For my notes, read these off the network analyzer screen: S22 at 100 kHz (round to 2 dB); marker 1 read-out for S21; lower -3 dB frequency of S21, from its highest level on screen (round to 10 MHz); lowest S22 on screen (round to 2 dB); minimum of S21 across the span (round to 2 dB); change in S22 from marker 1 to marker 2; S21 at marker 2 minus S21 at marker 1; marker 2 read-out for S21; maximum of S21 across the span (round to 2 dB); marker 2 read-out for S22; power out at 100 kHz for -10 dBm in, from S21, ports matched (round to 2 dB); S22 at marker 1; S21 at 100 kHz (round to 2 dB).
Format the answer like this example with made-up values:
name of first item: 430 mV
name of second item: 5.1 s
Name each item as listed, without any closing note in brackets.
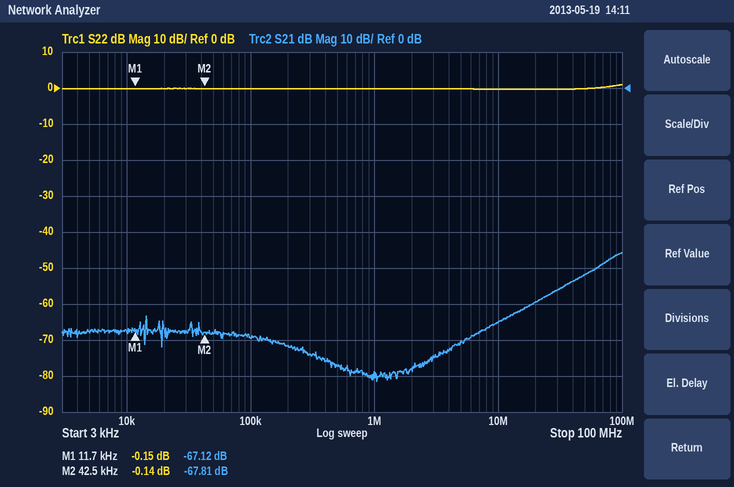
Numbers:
S22 at 100 kHz: 0 dB
marker 1 read-out for S21: -67.12 dB
lower -3 dB frequency of S21, from its highest level on screen: 70 MHz
lowest S22 on screen: 0 dB
minimum of S21 across the span: -82 dB
change in S22 from marker 1 to marker 2: 0.01 dB
S21 at marker 2 minus S21 at marker 1: -0.69 dB
marker 2 read-out for S21: -67.81 dB
maximum of S21 across the span: -46 dB
marker 2 read-out for S22: -0.14 dB
power out at 100 kHz for -10 dBm in, from S21, ports matched: -80 dBm
S22 at marker 1: -0.15 dB
S21 at 100 kHz: -70 dB
